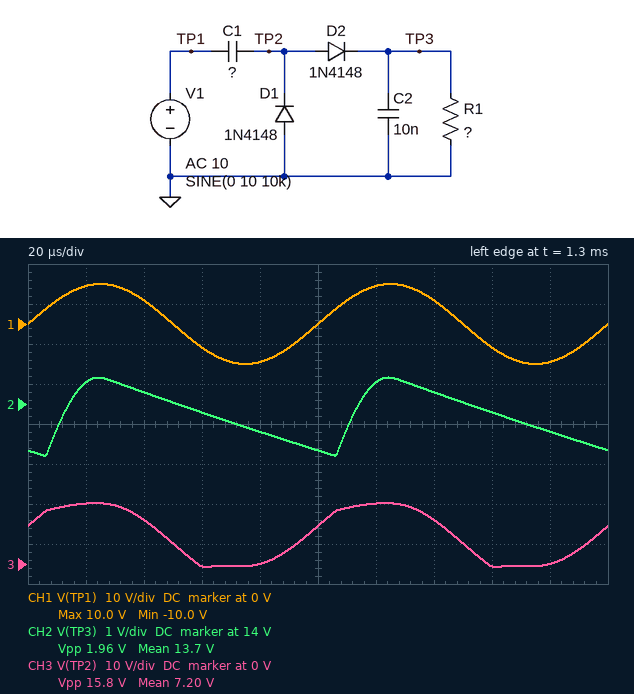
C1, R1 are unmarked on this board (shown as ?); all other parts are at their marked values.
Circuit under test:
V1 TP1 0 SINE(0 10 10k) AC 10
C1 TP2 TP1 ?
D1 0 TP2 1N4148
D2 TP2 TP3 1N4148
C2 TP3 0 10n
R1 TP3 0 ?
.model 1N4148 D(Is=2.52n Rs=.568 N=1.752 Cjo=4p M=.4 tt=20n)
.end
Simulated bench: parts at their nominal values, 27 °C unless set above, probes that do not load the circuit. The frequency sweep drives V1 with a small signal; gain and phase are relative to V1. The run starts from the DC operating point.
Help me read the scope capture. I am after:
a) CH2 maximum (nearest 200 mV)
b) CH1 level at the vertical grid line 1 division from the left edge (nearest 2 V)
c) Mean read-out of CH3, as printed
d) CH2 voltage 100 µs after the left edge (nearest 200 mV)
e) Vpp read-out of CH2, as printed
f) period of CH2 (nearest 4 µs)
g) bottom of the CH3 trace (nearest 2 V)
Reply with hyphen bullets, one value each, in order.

- 14.6 V
- 10 V
- 7.20 V
- 12.8 V
- 1.96 V
- 100 µs
- 0 V
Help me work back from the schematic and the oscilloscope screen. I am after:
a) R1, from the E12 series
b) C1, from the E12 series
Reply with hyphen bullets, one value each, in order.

- 56 kΩ
- 5.6 nF
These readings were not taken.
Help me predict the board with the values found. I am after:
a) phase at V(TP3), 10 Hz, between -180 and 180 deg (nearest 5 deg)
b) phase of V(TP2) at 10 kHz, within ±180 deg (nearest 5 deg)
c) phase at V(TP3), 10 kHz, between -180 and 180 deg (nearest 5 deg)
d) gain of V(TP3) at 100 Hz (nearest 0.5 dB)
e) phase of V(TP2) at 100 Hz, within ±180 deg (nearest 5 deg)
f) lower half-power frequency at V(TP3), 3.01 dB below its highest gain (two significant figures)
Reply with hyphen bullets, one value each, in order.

- 15 deg
- 0 deg
- -10 deg
- -50.5 dB
- 0 deg
- 3.1 Hz
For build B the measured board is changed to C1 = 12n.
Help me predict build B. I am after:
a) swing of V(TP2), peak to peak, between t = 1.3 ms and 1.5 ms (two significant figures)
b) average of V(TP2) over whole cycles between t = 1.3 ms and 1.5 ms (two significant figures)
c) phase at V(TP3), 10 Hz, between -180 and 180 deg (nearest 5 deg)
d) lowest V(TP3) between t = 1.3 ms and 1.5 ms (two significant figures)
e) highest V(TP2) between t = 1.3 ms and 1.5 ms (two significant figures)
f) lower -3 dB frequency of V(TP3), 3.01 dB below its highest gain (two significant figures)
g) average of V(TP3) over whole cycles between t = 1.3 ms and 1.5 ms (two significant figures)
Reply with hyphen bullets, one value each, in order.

- 18 V
- 8.3 V
- 5 deg
- 14 V
- 17 V
- 1.5 Hz
- 16 V
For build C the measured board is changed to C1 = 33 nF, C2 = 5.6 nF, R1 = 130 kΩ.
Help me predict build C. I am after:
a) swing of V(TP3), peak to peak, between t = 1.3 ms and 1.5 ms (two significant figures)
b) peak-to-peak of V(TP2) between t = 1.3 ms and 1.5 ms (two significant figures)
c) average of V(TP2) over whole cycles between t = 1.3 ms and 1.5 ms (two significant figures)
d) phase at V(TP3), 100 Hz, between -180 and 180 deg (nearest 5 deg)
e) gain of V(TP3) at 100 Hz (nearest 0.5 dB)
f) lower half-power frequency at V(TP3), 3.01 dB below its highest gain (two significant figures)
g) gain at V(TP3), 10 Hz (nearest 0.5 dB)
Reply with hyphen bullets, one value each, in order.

- 2.1 V
- 20 V
- 9.2 V
- -20 deg
- -43.5 dB
- 530 mHz
- -43.0 dB
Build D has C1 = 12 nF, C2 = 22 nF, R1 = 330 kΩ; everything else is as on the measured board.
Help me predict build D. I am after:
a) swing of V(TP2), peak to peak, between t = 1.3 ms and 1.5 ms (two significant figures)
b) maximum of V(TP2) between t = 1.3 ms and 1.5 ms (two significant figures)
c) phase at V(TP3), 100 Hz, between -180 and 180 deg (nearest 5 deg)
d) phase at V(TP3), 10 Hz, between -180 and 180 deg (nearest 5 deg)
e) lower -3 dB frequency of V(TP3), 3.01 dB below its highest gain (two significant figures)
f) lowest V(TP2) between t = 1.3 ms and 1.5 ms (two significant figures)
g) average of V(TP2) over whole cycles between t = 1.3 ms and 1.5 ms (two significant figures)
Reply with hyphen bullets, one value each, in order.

- 20 V
- 19 V
- -75 deg
- -15 deg
- 1.3 Hz
- -610 mV
- 9.2 V
